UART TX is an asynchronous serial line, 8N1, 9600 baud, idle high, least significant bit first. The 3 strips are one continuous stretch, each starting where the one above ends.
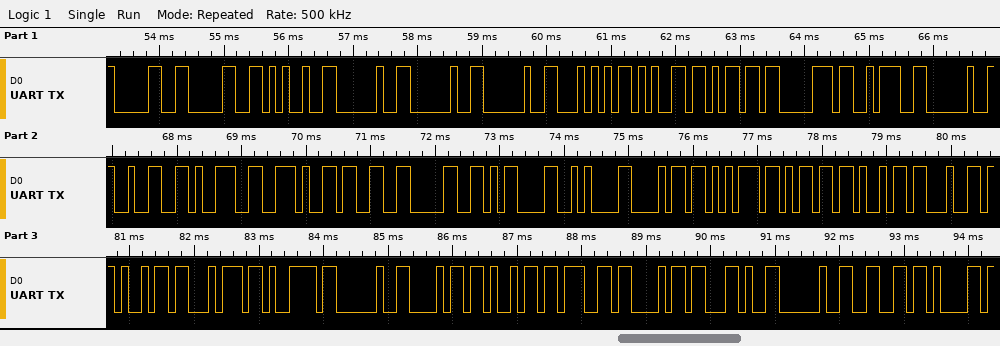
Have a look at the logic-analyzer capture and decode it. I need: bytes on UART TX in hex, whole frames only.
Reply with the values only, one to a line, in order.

30 30 25 20 20 20 54 65 6D 70 3A 20 32 39 2E 33 30 0D 0A 68 75 6D 69 64 69 74 79 20 68 69 67 68 2C 20 66 61
